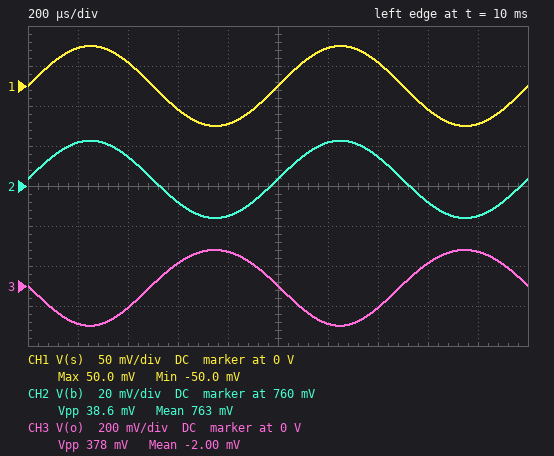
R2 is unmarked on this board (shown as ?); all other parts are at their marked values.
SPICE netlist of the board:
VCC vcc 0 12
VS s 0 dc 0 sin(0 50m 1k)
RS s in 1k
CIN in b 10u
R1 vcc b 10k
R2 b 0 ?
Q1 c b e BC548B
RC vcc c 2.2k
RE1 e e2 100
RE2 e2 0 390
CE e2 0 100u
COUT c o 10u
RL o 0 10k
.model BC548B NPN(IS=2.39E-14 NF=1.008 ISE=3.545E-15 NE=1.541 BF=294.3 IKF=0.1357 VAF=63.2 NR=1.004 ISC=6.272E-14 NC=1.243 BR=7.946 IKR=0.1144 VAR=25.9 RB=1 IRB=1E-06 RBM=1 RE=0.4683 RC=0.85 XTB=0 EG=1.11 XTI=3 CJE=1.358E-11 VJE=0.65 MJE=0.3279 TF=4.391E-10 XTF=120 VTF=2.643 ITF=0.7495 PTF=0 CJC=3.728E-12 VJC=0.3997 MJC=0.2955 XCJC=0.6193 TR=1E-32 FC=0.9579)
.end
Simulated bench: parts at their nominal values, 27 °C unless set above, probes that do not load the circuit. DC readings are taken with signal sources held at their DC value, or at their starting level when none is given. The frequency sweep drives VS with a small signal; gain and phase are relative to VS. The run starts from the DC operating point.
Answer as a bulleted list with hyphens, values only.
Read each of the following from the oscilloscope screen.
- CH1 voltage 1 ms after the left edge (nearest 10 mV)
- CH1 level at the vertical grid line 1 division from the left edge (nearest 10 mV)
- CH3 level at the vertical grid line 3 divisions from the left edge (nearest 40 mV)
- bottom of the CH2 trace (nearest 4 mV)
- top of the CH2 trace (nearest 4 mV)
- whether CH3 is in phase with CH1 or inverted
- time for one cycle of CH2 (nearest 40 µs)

- 0 V
- 50 mV
- 120 mV
- 744 mV
- 784 mV
- inverted
- 1.00 ms
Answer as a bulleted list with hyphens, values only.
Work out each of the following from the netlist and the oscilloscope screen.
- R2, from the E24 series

- 680 Ω
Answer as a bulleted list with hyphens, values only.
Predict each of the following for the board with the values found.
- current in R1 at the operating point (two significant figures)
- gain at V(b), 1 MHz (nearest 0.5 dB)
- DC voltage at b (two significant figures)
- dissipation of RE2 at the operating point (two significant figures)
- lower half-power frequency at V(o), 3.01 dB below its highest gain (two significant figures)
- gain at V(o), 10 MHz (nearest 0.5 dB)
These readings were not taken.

- 1.1 mA
- -8.5 dB
- 760 mV
- 41 µW
- 17 Hz
- 9.0 dB
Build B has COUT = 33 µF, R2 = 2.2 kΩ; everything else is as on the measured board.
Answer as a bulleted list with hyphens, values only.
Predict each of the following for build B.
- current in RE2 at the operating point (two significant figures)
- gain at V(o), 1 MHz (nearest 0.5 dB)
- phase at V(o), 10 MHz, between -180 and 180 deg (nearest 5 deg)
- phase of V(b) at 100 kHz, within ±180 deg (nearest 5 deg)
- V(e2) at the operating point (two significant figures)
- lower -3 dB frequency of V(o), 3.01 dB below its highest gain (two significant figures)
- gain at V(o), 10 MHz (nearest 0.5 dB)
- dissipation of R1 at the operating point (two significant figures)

- 3.0 mA
- 20.0 dB
- 115 deg
- 0 deg
- 1.2 V
- 19 Hz
- 13.5 dB
- 9.7 mW
